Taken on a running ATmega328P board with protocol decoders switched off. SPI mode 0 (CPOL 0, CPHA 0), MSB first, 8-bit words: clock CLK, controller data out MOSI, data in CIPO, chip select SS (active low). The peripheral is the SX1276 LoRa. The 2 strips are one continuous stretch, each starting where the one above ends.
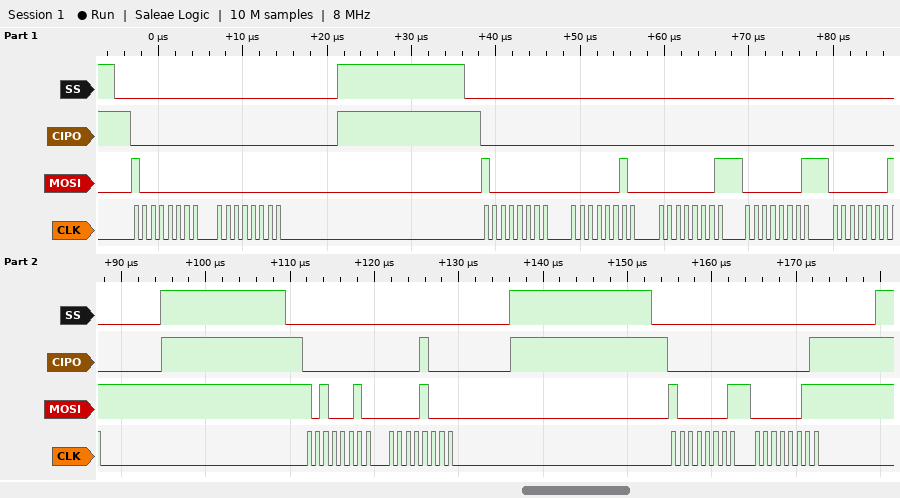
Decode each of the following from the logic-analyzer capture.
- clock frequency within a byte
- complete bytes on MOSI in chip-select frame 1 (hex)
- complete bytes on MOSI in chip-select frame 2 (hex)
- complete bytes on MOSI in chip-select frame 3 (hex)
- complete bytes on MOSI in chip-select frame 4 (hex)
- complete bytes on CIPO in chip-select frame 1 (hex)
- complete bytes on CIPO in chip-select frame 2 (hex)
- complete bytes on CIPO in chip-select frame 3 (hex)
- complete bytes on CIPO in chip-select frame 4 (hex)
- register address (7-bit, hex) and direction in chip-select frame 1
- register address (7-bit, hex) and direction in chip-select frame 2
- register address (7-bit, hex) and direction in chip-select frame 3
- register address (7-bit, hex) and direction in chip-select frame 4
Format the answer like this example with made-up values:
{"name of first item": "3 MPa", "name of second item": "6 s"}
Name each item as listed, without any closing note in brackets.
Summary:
{"clock frequency within a byte": "1 MHz", "complete bytes on MOSI in chip-select frame 1": "80 00", "complete bytes on MOSI in chip-select frame 2": "80 02 01 01 01", "complete bytes on MOSI in chip-select frame 3": "A2 08", "complete bytes on MOSI in chip-select frame 4": "81 03", "complete bytes on CIPO in chip-select frame 1": "00 00", "complete bytes on CIPO in chip-select frame 2": "00 00 00 00 00", "complete bytes on CIPO in chip-select frame 3": "00 08", "complete bytes on CIPO in chip-select frame 4": "00 01", "register address (7-bit, hex) and direction in chip-select frame 1": "0x00 write", "register address (7-bit, hex) and direction in chip-select frame 2": "0x00 write", "register address (7-bit, hex) and direction in chip-select frame 3": "0x22 write", "register address (7-bit, hex) and direction in chip-select frame 4": "0x01 write"}
